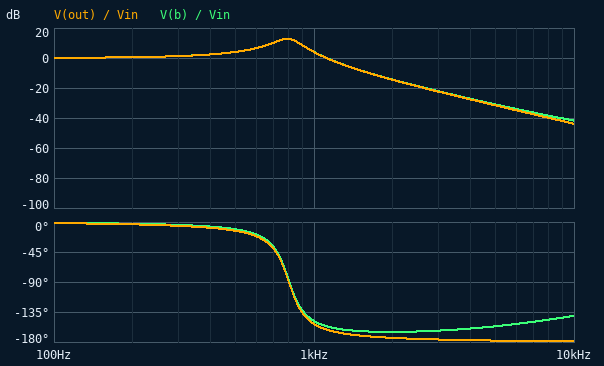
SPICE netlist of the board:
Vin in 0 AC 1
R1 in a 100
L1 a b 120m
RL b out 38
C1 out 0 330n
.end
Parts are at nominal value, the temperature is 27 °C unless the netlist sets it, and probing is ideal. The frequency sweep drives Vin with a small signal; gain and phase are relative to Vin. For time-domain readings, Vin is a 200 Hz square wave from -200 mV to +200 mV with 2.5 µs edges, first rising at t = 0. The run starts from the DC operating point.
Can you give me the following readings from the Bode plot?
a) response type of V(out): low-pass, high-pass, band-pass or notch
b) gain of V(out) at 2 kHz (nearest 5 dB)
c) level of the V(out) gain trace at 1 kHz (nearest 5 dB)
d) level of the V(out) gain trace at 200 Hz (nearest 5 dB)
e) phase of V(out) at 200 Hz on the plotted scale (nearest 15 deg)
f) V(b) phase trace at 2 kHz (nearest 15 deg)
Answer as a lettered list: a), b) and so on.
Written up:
a) low-pass
b) -15 dB
c) 5 dB
d) 0 dB
e) 0 deg
f) -165 deg
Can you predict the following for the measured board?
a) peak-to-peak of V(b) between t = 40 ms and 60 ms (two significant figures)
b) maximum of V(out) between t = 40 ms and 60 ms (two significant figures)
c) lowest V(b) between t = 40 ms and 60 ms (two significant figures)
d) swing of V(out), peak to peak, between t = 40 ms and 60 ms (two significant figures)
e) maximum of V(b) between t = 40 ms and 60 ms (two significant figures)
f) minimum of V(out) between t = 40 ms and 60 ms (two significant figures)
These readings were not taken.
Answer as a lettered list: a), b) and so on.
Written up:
a) 850 mV
b) 430 mV
c) -430 mV
d) 850 mV
e) 430 mV
f) -430 mV
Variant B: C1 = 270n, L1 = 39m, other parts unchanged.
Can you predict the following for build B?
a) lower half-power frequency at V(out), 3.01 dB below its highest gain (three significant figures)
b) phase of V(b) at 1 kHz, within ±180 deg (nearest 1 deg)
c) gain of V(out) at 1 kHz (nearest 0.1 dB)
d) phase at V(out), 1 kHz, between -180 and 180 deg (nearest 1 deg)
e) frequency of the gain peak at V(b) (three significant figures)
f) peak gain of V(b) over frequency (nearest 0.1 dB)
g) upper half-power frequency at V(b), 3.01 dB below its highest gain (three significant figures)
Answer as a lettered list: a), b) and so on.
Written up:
a) 1.18 kHz
b) -18 deg
c) 4.0 dB
d) -22 deg
e) 1.50 kHz
f) 9.0 dB
g) 1.76 kHz
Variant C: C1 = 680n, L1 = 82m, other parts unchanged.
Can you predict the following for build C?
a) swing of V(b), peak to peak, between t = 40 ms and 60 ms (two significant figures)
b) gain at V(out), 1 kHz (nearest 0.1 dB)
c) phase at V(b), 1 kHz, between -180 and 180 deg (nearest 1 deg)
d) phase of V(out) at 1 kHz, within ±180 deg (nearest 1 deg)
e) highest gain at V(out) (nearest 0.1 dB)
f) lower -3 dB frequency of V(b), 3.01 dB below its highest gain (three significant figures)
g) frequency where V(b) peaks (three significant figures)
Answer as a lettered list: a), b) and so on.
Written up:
a) 870 mV
b) -2.5 dB
c) -145 deg
d) -154 deg
e) 8.2 dB
f) 492 Hz
g) 647 Hz
